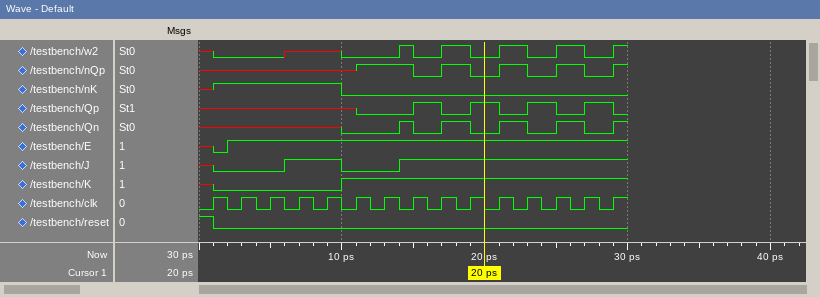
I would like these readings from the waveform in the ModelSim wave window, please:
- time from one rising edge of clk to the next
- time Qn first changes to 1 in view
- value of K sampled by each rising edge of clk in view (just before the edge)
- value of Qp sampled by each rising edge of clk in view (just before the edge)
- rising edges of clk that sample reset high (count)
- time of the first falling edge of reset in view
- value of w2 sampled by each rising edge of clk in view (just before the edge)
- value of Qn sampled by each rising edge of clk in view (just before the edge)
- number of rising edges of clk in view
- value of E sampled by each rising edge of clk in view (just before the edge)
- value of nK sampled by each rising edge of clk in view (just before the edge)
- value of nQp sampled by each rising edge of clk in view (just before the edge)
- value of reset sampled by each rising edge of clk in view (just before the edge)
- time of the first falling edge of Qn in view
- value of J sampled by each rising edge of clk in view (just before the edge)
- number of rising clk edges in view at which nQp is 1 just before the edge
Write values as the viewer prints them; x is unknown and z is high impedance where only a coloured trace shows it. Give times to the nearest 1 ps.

2 ps
14 ps
x 0 0 0 0 1 1 1 1 1 1 1 1 1 1
x x x x x x 0 0 1 0 1 0 1 0 1
1
1 ps
x 0 0 x x 0 0 1 0 1 0 1 0 1 0
x x x x x 0 0 1 0 1 0 1 0 1 0
15
x 1 1 1 1 1 1 1 1 1 1 1 1 1 1
x 1 1 1 1 0 0 0 0 0 0 0 0 0 0
x x x x x x 1 1 0 1 0 1 0 1 0
1 0 0 0 0 0 0 0 0 0 0 0 0 0 0
15 ps
x 0 0 1 1 0 0 1 1 1 1 1 1 1 1
5
